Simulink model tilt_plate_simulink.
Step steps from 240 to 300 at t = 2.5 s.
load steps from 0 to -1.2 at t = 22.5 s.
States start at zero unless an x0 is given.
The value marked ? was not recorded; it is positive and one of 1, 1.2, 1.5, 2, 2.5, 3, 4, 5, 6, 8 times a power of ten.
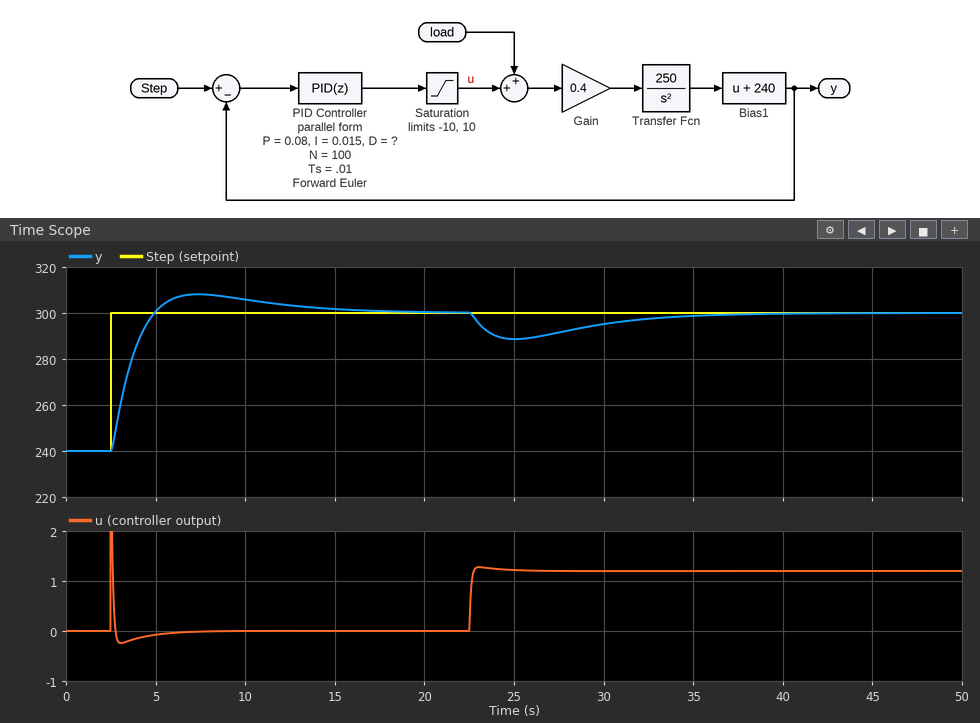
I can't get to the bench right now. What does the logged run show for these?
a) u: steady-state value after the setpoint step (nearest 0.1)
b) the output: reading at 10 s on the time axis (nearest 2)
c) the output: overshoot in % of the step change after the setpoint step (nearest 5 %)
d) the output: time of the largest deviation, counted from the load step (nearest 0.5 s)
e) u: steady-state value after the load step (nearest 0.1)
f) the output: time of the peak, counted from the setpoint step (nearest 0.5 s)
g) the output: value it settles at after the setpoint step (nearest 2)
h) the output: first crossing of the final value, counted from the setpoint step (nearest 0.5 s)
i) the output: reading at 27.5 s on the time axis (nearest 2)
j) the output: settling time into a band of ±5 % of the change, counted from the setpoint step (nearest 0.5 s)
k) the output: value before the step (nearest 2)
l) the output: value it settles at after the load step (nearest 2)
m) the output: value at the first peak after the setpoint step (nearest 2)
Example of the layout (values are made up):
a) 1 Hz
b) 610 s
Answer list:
a) 0.0
b) 306
c) 15 %
d) 2.5 s
e) 1.2
f) 5.0 s
g) 300
h) 2.5 s
i) 292
j) 10.5 s
k) 240
l) 300
m) 308
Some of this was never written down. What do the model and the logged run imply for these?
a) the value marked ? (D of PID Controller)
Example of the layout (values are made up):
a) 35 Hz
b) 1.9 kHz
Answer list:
a) 0.1
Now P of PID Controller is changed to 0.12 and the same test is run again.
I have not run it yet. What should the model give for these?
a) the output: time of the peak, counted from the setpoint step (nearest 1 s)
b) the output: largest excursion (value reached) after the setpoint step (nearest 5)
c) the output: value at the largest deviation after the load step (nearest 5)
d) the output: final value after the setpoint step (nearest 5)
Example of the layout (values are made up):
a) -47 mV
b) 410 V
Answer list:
a) 4 s
b) 305
c) 290
d) 300
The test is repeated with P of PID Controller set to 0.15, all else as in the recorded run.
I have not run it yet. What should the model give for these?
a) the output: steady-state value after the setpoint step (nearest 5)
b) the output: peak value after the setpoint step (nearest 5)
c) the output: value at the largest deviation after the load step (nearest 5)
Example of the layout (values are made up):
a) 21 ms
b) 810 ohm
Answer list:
a) 300
b) 305
c) 295
